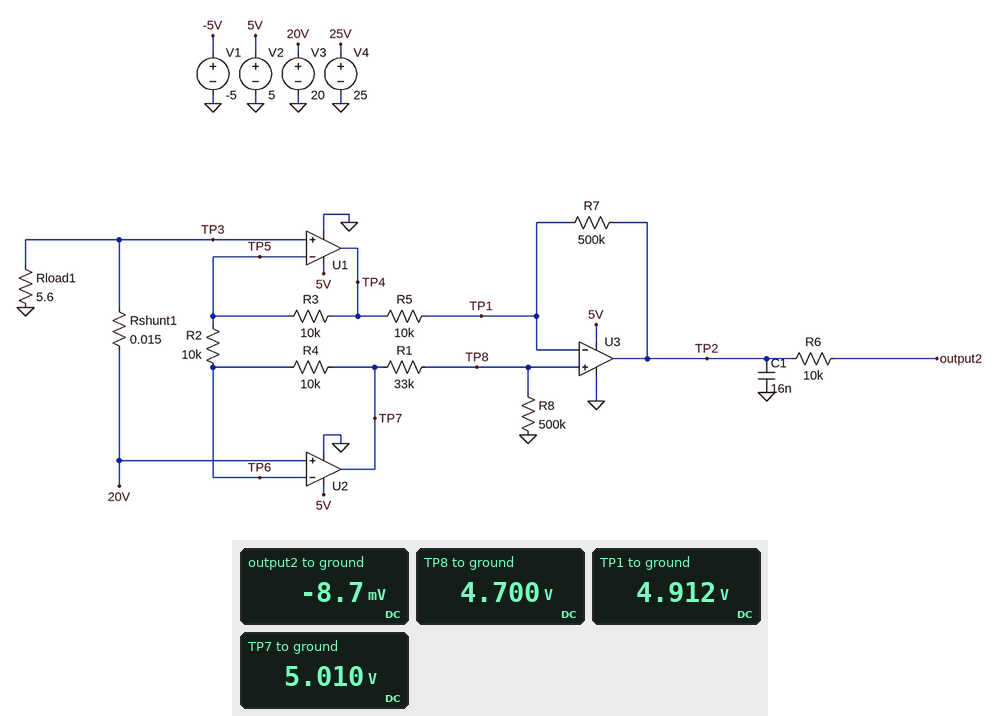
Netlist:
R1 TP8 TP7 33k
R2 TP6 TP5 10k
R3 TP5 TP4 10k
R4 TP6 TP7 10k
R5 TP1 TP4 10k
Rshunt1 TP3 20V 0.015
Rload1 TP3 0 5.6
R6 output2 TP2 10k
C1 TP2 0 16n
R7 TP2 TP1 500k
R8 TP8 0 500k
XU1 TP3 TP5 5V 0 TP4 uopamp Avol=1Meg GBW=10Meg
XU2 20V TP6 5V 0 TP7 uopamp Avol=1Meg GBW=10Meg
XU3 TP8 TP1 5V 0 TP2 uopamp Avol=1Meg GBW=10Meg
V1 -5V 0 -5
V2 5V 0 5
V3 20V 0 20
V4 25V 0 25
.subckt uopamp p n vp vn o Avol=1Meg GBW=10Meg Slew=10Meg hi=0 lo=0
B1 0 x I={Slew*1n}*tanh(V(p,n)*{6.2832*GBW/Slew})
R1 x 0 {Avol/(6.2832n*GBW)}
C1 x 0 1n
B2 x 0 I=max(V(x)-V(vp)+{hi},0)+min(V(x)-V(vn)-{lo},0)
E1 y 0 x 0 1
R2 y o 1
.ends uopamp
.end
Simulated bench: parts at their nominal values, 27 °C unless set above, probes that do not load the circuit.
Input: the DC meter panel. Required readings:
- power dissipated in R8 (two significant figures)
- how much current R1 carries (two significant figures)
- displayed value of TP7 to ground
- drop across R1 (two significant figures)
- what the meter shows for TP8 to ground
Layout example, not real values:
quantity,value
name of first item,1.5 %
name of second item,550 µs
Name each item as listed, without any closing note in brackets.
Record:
quantity,value
power dissipated in R8,44 µW
how much current R1 carries,9.4 µA
displayed value of TP7 to ground,5.010 V
drop across R1,310 mV
what the meter shows for TP8 to ground,4.700 V
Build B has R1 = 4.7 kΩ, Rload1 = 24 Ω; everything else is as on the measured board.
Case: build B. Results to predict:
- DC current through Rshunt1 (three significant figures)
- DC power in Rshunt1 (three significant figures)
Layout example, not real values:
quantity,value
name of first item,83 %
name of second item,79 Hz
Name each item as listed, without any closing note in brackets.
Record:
quantity,value
DC current through Rshunt1,833 mA
DC power in Rshunt1,10.4 mW
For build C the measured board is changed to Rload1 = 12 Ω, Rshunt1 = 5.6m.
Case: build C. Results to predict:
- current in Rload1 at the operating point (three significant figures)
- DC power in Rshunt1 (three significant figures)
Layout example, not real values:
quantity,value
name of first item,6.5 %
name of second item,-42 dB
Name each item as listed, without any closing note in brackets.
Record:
quantity,value
current in Rload1 at the operating point,1.67 A
DC power in Rshunt1,15.5 mW
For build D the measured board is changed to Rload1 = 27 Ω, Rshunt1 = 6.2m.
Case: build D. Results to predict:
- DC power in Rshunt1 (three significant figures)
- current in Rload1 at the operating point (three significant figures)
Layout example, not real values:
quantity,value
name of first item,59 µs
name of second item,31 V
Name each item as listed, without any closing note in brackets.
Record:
quantity,value
DC power in Rshunt1,3.40 mW
current in Rload1 at the operating point,741 mA
